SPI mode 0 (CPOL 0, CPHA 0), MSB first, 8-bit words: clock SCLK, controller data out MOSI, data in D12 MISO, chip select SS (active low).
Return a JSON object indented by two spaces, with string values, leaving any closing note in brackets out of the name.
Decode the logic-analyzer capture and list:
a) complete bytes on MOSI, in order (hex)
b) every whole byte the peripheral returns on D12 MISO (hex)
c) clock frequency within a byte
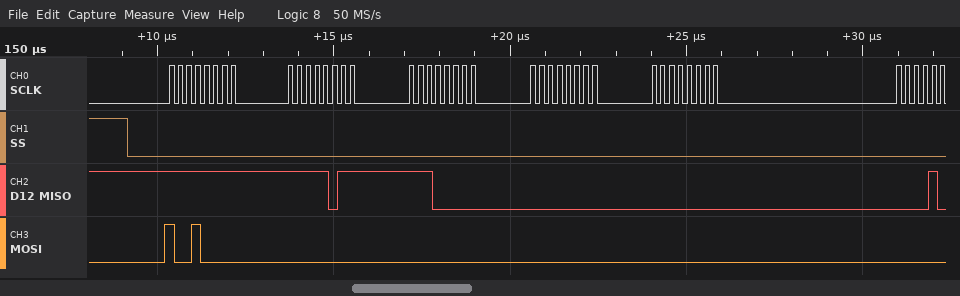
{
  "complete bytes on MOSI, in order": "90 00 00 00 00",
  "every whole byte the peripheral returns on D12 MISO": "FF FB E0 00 00",
  "clock frequency within a byte": "4 MHz"
}
